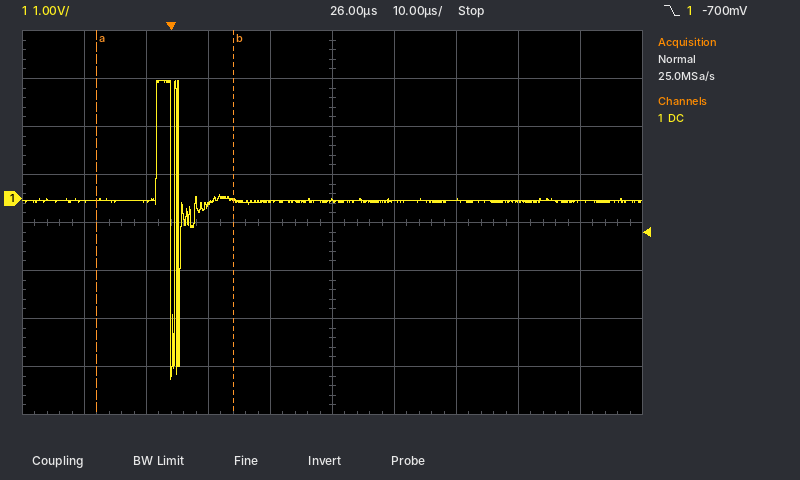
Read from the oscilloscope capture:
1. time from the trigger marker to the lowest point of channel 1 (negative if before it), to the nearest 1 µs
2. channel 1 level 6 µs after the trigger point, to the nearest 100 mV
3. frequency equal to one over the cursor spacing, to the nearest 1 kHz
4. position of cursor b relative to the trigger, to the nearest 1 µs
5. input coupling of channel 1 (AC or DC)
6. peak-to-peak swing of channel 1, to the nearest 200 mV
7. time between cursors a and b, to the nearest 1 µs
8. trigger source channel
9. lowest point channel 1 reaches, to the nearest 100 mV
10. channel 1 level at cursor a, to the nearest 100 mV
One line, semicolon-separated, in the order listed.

0 µs; -100 mV; 45 kHz; +10 µs; DC; 6.2 V; 22 µs; channel 1; -3.8 V; 0.0 V
